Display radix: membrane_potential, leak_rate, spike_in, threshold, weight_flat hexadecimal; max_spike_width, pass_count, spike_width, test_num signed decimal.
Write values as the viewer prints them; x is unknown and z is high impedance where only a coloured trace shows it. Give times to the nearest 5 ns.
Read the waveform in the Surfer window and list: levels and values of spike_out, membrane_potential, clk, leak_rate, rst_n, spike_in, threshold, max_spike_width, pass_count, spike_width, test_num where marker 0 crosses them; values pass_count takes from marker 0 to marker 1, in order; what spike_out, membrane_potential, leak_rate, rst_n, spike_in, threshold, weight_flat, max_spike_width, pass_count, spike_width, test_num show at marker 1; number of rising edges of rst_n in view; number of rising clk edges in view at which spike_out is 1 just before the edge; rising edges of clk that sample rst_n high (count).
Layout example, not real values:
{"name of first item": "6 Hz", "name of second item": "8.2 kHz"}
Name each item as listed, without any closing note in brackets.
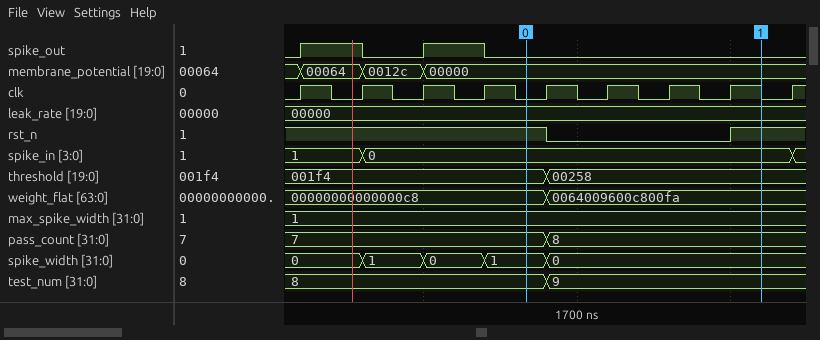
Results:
{"levels and values of spike_out, membrane_potential, clk, leak_rate, rst_n, spike_in, threshold, max_spike_width, pass_count, spike_width, test_num where marker 0 crosses them": "spike_out=0, membrane_potential=00000, clk=0, leak_rate=00000, rst_n=1, spike_in=0, threshold=001f4, max_spike_width=1, pass_count=7, spike_width=1, test_num=8", "values pass_count takes from marker 0 to marker 1, in order": "7, 8", "what spike_out, membrane_potential, leak_rate, rst_n, spike_in, threshold, weight_flat, max_spike_width, pass_count, spike_width, test_num show at marker 1": "spike_out=0, membrane_potential=00000, leak_rate=00000, rst_n=1, spike_in=0, threshold=00258, weight_flat=0064009600c800fa, max_spike_width=1, pass_count=8, spike_width=0, test_num=9", "number of rising edges of rst_n in view": "1", "number of rising clk edges in view at which spike_out is 1 just before the edge": "2", "rising edges of clk that sample rst_n high": "6"}
